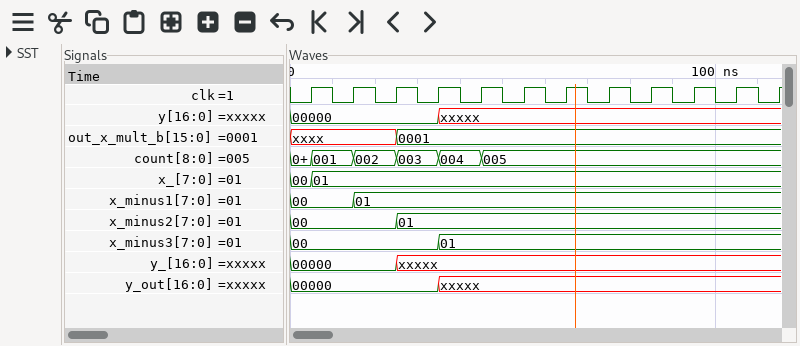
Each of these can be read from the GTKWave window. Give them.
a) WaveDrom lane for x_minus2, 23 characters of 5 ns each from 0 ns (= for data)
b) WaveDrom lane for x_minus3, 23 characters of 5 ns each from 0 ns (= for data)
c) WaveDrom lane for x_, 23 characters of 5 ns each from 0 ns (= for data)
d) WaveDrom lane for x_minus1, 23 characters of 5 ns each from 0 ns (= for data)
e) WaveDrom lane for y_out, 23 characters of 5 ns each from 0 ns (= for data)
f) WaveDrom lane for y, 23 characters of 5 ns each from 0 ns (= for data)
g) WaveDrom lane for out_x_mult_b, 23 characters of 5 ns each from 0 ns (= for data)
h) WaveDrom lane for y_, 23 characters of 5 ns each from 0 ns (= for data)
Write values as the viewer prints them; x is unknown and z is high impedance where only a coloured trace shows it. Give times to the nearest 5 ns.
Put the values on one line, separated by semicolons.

{name: 'x_minus2', wave: '=....=.................', data: '00 01'}; {name: 'x_minus3', wave: '=......=...............', data: '00 01'}; {name: 'x_', wave: '==.....................', data: '00 01'}; {name: 'x_minus1', wave: '=..=...................', data: '00 01'}; {name: 'y_out', wave: '=......x...............', data: '00000'}; {name: 'y', wave: '=......x...............', data: '00000'}; {name: 'out_x_mult_b', wave: 'x....=.................', data: '0001'}; {name: 'y_', wave: '=....x.................', data: '00000'}
